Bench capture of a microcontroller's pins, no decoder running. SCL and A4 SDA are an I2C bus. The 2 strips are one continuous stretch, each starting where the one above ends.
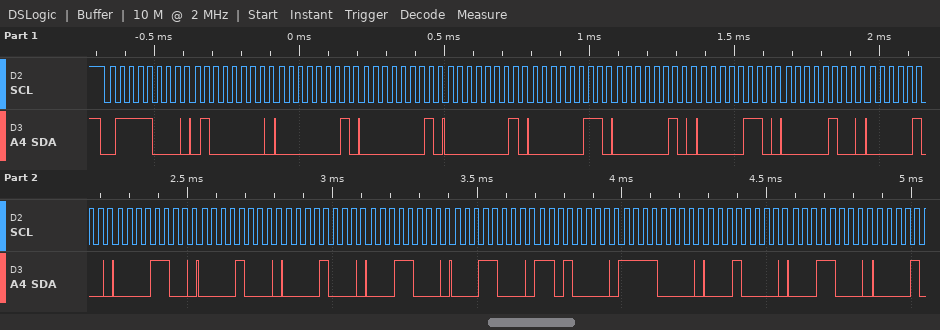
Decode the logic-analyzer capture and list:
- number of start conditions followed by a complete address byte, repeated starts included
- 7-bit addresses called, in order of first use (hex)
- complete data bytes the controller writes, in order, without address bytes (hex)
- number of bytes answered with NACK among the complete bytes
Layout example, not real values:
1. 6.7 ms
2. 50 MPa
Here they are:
1. 1
2. 0x3C
3. 40 01 01 01 03 02 06 04 04 0C 08 08 18 18 D0 F0 10 18
4. 0
